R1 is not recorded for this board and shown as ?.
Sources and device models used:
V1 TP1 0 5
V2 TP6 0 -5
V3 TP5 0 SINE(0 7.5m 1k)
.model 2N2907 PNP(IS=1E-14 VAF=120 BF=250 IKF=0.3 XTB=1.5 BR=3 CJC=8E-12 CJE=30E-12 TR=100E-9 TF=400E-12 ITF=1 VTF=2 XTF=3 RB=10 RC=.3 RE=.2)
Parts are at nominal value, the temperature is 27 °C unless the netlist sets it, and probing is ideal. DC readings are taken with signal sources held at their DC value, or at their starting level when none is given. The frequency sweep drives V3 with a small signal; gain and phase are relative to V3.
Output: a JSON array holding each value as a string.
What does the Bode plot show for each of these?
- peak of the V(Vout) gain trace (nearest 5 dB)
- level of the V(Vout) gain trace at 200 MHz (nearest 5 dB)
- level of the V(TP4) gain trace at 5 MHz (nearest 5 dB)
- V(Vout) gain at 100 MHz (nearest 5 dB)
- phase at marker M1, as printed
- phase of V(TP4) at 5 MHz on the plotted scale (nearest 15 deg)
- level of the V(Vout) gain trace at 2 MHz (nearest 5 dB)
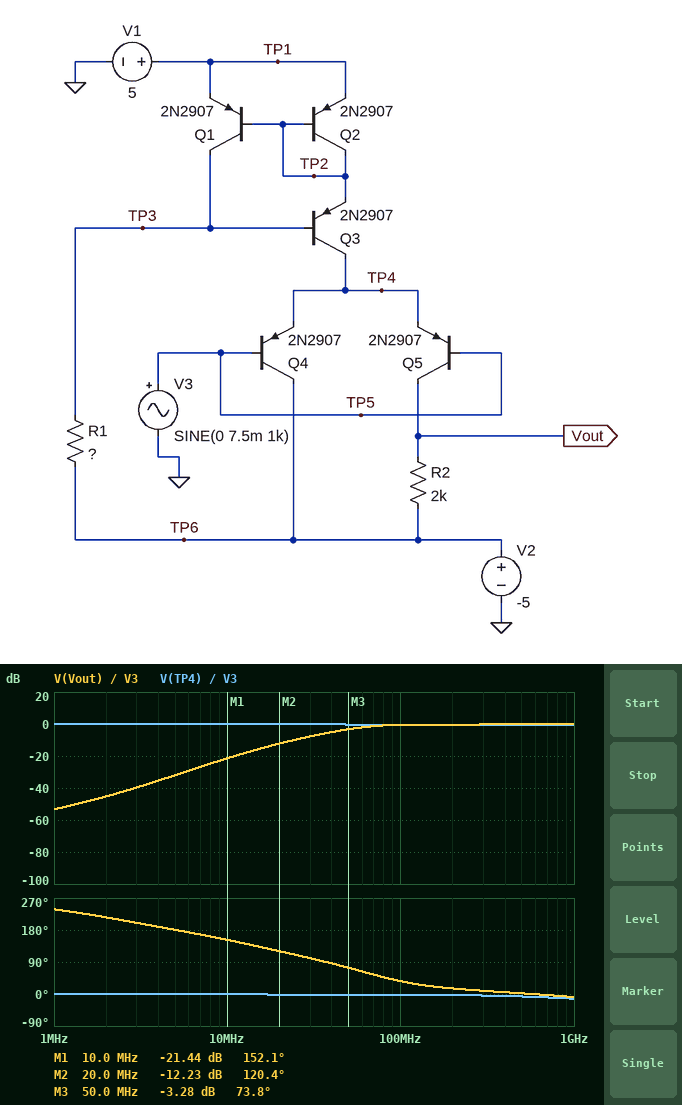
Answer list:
["0 dB", "0 dB", "0 dB", "0 dB", "152.1 deg", "0 deg", "-45 dB"]
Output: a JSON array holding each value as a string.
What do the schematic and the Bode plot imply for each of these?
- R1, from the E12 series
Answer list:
["6.8 kΩ"]
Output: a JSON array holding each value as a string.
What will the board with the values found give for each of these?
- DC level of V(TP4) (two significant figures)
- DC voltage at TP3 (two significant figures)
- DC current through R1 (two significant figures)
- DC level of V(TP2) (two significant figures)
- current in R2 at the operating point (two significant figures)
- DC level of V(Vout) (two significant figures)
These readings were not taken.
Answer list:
["640 mV", "3.7 V", "1.3 mA", "4.3 V", "630 µA", "-3.7 V"]
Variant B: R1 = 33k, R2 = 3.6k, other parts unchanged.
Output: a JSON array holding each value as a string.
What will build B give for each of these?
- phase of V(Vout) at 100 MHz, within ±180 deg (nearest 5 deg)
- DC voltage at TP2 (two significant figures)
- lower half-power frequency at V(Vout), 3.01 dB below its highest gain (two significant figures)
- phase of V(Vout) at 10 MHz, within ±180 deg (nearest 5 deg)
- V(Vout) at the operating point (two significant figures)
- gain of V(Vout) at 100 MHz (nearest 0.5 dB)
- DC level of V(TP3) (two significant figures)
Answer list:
["10 deg", "4.4 V", "15 MHz", "110 deg", "-4.5 V", "0 dB", "3.8 V"]
